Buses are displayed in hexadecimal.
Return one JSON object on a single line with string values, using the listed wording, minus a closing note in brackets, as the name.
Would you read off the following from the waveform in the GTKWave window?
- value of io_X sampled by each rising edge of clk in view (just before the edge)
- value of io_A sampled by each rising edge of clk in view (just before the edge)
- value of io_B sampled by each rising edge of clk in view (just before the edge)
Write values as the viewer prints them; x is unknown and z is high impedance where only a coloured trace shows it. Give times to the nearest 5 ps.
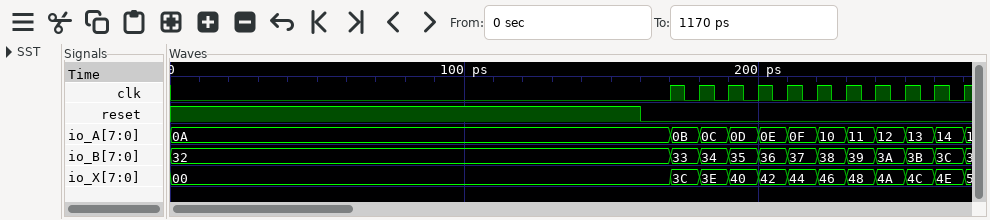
{"value of io_X sampled by each rising edge of clk in view": "00, 3C, 3E, 40, 42, 44, 46, 48, 4A, 4C, 4E", "value of io_A sampled by each rising edge of clk in view": "0A, 0B, 0C, 0D, 0E, 0F, 10, 11, 12, 13, 14", "value of io_B sampled by each rising edge of clk in view": "32, 33, 34, 35, 36, 37, 38, 39, 3A, 3B, 3C"}
